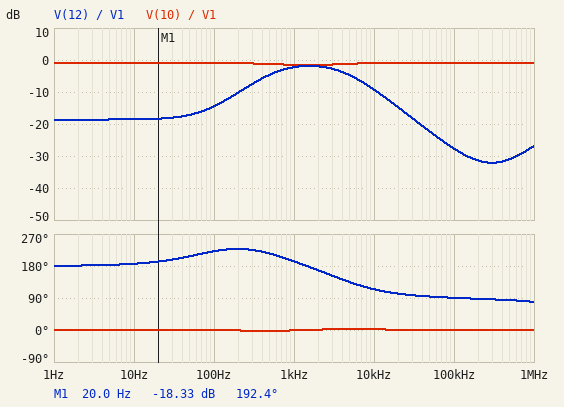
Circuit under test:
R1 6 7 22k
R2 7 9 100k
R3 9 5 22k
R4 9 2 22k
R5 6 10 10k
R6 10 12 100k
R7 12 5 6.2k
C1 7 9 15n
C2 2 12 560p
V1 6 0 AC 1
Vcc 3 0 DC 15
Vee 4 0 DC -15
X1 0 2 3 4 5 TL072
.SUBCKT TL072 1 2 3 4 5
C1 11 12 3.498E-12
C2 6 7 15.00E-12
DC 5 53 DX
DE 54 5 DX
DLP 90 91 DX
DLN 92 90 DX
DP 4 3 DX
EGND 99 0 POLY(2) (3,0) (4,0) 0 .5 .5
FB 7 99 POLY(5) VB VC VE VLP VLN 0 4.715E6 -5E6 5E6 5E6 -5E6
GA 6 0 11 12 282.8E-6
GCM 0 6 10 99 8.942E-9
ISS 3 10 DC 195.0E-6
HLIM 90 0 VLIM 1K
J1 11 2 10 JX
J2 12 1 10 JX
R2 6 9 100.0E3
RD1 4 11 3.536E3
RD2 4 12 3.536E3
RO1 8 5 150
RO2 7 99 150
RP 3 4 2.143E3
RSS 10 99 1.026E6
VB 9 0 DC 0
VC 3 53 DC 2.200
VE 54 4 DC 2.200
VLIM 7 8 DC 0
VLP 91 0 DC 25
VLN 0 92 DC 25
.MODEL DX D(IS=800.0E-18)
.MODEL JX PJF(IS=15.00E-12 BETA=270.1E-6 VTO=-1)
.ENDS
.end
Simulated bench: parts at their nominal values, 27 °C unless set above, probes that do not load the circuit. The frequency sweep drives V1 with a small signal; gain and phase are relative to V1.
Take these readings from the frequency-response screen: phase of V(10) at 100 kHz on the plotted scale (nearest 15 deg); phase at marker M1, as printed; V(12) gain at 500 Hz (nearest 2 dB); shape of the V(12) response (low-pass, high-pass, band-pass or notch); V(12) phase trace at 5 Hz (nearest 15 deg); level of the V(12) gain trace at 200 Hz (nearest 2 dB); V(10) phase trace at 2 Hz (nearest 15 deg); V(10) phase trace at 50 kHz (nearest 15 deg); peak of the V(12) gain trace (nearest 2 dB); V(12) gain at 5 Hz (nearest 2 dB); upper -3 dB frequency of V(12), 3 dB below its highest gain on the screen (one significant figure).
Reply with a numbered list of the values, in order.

1. 0 deg
2. 192.4 deg
3. -4 dB
4. band-pass
5. 180 deg
6. -10 dB
7. 0 deg
8. 0 deg
9. -2 dB
10. -18 dB
11. 5 kHz
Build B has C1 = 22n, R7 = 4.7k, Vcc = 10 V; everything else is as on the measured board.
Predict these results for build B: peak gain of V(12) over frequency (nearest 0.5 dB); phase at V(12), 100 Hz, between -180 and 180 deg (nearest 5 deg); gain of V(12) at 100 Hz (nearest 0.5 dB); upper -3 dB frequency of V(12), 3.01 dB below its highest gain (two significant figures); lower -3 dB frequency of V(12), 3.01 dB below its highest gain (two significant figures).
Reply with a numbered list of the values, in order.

1. -1.5 dB
2. -135 deg
3. -12.0 dB
4. 4.8 kHz
5. 340 Hz
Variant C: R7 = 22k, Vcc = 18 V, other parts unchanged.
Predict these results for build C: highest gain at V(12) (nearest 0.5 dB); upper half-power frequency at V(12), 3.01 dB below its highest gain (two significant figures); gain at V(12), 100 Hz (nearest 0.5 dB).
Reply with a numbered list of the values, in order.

1. -4.5 dB
2. 4.8 kHz
3. -19.0 dB
